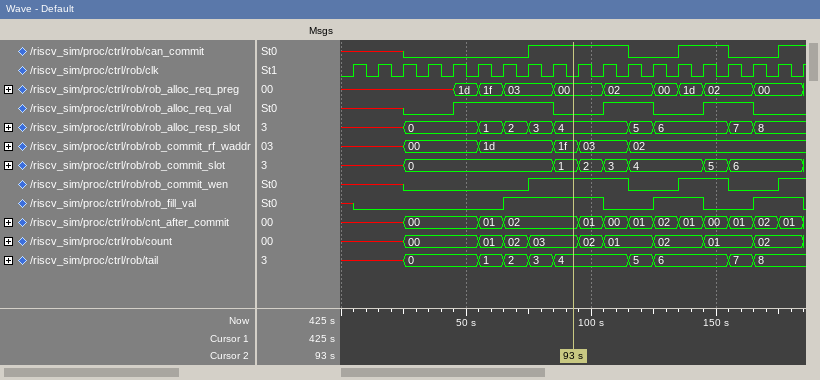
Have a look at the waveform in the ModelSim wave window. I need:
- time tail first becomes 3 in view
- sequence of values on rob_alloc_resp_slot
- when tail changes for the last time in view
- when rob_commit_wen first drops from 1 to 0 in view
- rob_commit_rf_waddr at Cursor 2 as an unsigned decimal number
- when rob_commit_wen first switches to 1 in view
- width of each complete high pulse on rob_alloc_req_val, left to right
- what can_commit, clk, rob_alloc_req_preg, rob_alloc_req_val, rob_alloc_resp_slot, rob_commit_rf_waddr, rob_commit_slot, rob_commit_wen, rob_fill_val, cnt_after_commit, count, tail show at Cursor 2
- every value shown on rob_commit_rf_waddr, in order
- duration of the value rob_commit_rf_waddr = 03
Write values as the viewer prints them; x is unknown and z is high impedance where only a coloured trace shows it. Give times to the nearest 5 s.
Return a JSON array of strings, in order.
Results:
["75 s", "x, 0, 1, 2, 3, 4, 5, 6, 7, 8", "165 s", "115 s", "31", "75 s", "40 s, 20 s, 20 s", "can_commit=1, clk=0, rob_alloc_req_preg=00, rob_alloc_req_val=0, rob_alloc_resp_slot=4, rob_commit_rf_waddr=1f, rob_commit_slot=1, rob_commit_wen=1, rob_fill_val=1, cnt_after_commit=02, count=03, tail=4", "x, 00, 1d, 1f, 03, 02", "20 s"]
